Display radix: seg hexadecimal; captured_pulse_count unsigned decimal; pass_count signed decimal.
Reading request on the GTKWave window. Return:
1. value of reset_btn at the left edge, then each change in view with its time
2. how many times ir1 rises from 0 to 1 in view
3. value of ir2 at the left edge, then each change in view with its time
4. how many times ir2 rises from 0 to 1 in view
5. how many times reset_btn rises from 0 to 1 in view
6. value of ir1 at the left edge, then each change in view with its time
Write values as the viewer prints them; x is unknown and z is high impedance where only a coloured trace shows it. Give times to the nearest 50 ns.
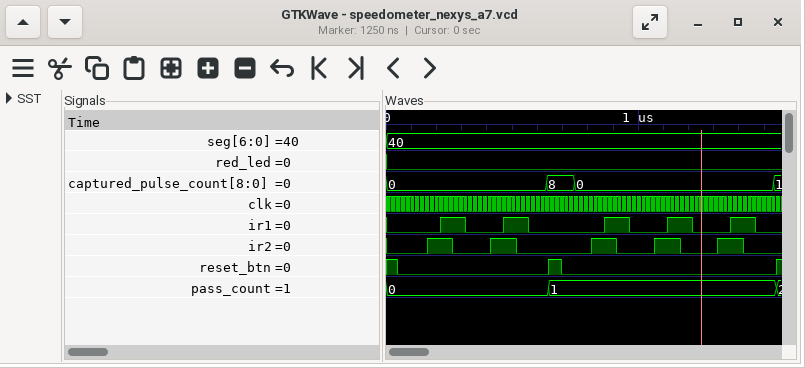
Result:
1, 0 at 50 ns, 1 at 650 ns, 0 at 700 ns, 1 at 1550 ns
5
0, 1 at 150 ns, 0 at 250 ns, 1 at 400 ns, 0 at 500 ns, 1 at 800 ns, 0 at 900 ns, 1 at 1050 ns, 0 at 1150 ns, 1 at 1300 ns, 0 at 1400 ns
5
2
0, 1 at 200 ns, 0 at 300 ns, 1 at 450 ns, 0 at 550 ns, 1 at 850 ns, 0 at 950 ns, 1 at 1100 ns, 0 at 1200 ns, 1 at 1350 ns, 0 at 1450 ns
